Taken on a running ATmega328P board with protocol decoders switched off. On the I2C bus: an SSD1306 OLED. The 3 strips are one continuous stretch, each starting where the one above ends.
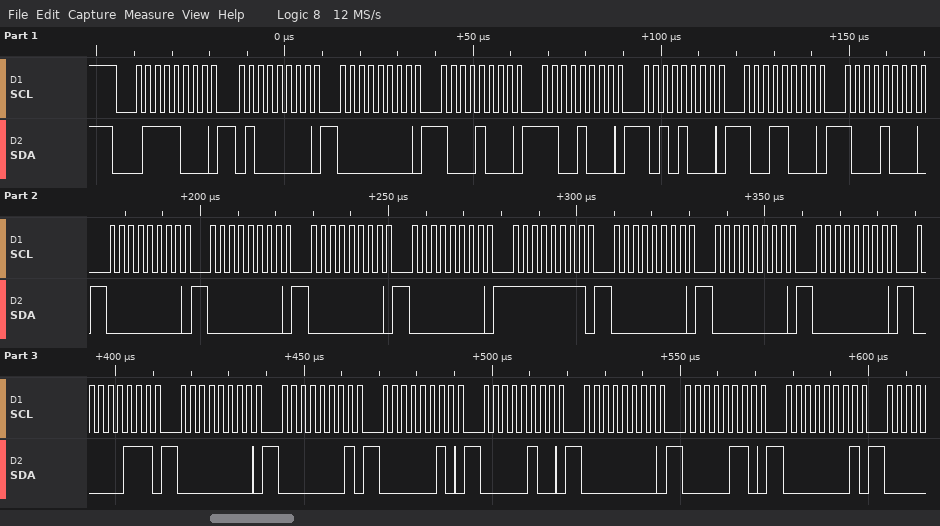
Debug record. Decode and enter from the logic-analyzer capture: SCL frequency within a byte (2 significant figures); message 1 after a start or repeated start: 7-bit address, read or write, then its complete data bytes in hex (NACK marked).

400 kHz
0x3C write: 40 00 88 C8 A8 98 88 00 00 00 00 FF 00 00 00 07 00 01 02 04 00 06 01
